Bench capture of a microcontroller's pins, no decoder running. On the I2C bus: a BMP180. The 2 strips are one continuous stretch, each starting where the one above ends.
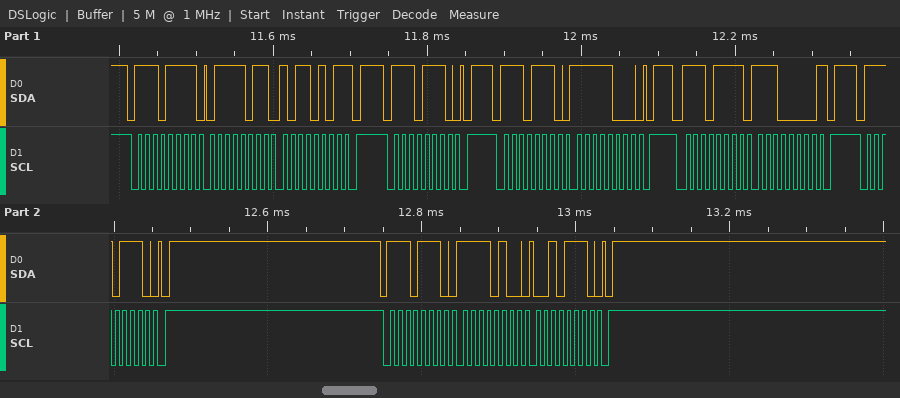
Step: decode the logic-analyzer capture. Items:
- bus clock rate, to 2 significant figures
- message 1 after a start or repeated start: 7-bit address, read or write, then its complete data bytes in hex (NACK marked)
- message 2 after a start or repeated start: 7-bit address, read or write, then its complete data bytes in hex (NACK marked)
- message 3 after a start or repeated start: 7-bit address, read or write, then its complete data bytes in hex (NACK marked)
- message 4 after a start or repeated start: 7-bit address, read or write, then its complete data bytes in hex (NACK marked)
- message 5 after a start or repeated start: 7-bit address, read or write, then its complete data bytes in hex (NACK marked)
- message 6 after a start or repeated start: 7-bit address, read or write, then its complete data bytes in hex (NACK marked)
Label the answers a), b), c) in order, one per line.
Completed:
a) 100 kHz
b) 0x77 read: 7B B5 NACK
c) 0x77 write
d) 0x77 write: F8
e) 0x77 read: E0 NACK
f) 0x77 write
g) 0x77 write: F4 2E
